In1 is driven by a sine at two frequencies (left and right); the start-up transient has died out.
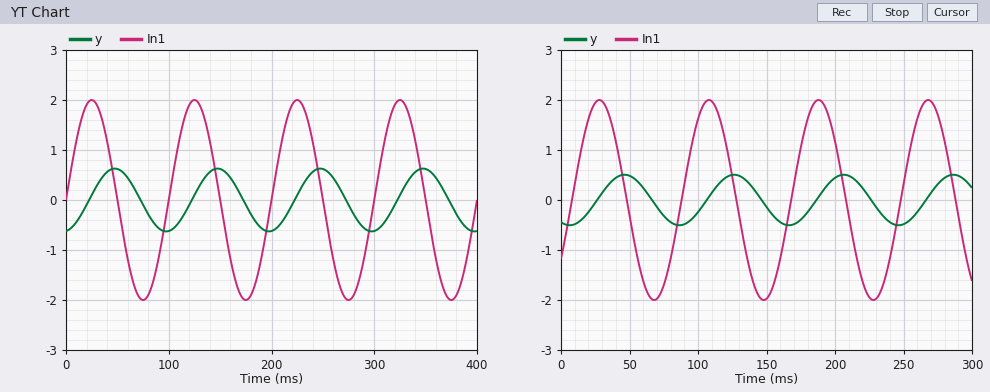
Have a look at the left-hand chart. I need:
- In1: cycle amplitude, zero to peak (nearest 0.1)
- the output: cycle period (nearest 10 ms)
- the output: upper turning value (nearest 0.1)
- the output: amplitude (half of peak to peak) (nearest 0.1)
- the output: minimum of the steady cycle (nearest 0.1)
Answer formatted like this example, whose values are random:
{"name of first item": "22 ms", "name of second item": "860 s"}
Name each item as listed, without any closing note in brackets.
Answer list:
{"In1: cycle amplitude, zero to peak": "2.0", "the output: cycle period": "100 ms", "the output: upper turning value": "0.6", "the output: amplitude (half of peak to peak)": "0.6", "the output: minimum of the steady cycle": "-0.6"}
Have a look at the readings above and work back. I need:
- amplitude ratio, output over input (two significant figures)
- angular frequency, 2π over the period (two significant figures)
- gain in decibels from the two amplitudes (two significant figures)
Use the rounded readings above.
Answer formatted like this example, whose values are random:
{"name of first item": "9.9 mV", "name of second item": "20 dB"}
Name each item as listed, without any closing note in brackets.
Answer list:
{"amplitude ratio, output over input": "0.30", "angular frequency, 2π over the period": "0.063 rad/ms", "gain in decibels from the two amplitudes": "-10 dB"}
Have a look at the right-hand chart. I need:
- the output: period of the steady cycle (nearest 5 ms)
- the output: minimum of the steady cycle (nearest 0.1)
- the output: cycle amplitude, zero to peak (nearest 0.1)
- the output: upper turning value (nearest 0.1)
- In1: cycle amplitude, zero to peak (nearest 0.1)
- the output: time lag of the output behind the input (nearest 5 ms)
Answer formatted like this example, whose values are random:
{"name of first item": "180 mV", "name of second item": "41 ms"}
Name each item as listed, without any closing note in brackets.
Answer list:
{"the output: period of the steady cycle": "80 ms", "the output: minimum of the steady cycle": "-0.5", "the output: cycle amplitude, zero to peak": "0.5", "the output: upper turning value": "0.5", "In1: cycle amplitude, zero to peak": "2.0", "the output: time lag of the output behind the input": "20 ms"}
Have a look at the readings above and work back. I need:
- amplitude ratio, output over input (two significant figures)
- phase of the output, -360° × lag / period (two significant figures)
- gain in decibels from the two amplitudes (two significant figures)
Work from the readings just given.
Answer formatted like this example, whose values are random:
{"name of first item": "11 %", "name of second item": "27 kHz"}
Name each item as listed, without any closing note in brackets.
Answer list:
{"amplitude ratio, output over input": "0.25", "phase of the output, -360° × lag / period": "-90°", "gain in decibels from the two amplitudes": "-12 dB"}
